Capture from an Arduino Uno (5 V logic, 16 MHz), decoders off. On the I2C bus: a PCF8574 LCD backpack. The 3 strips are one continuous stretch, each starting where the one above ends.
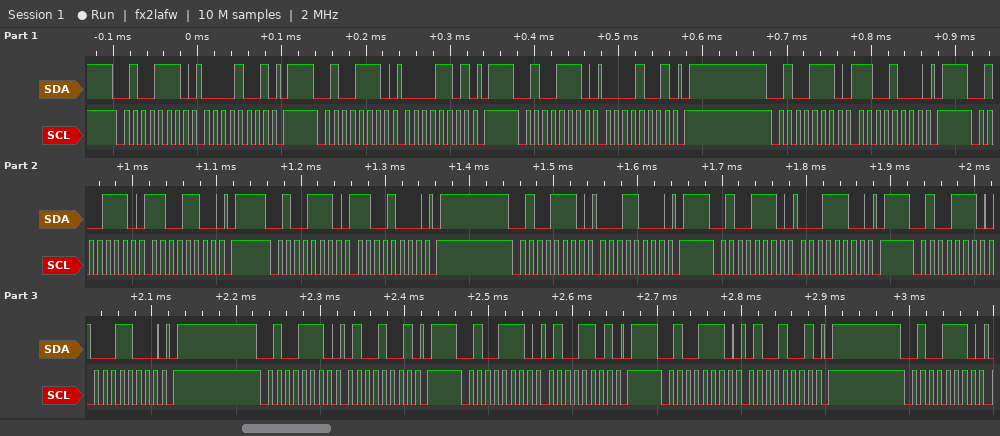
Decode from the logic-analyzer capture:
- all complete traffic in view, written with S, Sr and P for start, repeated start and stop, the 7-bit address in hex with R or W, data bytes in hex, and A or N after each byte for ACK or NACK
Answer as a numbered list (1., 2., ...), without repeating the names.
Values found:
1. S 27W A 09 A P S 27W A 0D A P S 27W A 09 A P S 27W A C8 A P S 27W A CC A P S 27W A C8 A P S 27W A 18 A P S 27W A 1C A P S 27W A 18 A P S 27W A 49 A P S 27W A 4D A P S 27W A 49 A P S 27W A
